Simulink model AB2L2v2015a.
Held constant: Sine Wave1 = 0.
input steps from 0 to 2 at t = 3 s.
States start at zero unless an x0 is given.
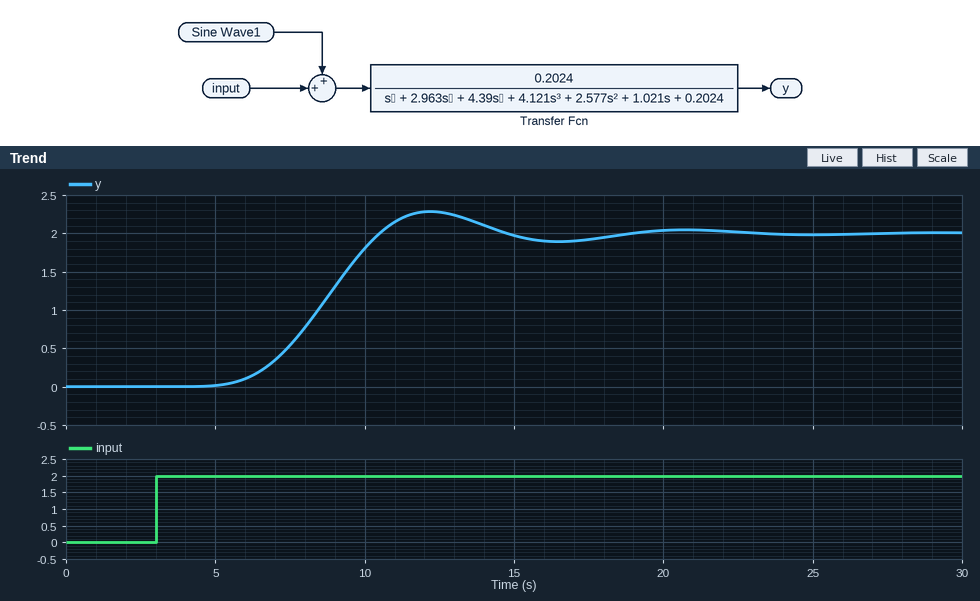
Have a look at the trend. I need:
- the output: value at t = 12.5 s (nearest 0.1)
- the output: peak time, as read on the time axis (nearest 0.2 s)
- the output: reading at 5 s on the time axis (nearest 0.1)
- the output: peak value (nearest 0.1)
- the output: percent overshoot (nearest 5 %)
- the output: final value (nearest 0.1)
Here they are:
2.3
12.2 s
0.0
2.3
15 %
2.0
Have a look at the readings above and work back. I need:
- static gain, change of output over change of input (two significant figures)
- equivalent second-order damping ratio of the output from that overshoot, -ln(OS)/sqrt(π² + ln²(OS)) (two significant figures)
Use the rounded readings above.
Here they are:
1.0
0.52
